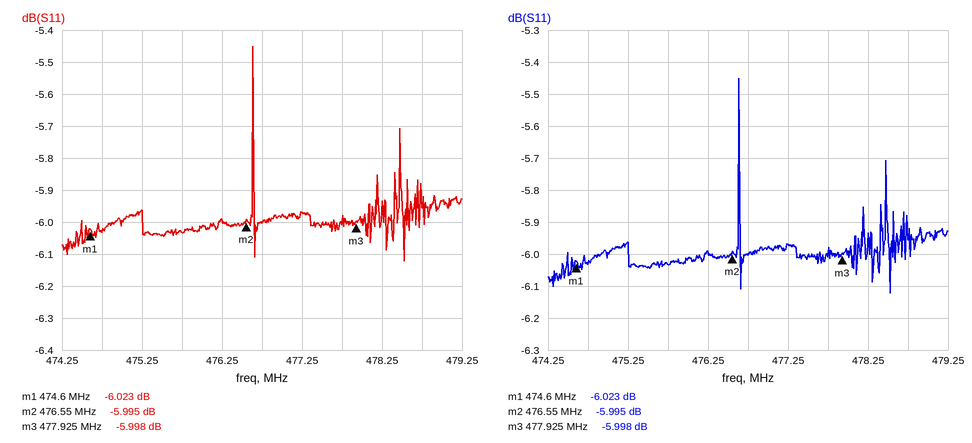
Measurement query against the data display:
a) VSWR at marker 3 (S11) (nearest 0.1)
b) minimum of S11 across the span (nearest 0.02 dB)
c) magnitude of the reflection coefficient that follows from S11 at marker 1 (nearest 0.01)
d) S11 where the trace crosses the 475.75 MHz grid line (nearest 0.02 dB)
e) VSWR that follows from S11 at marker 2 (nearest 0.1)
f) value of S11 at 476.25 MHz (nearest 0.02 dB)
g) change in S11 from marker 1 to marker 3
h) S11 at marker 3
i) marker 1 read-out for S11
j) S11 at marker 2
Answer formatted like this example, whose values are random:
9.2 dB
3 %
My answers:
3.0
-6.12 dB
0.50
-6.04 dB
3.0
-6.00 dB
0.025 dB
-5.998 dB
-6.023 dB
-5.995 dB
